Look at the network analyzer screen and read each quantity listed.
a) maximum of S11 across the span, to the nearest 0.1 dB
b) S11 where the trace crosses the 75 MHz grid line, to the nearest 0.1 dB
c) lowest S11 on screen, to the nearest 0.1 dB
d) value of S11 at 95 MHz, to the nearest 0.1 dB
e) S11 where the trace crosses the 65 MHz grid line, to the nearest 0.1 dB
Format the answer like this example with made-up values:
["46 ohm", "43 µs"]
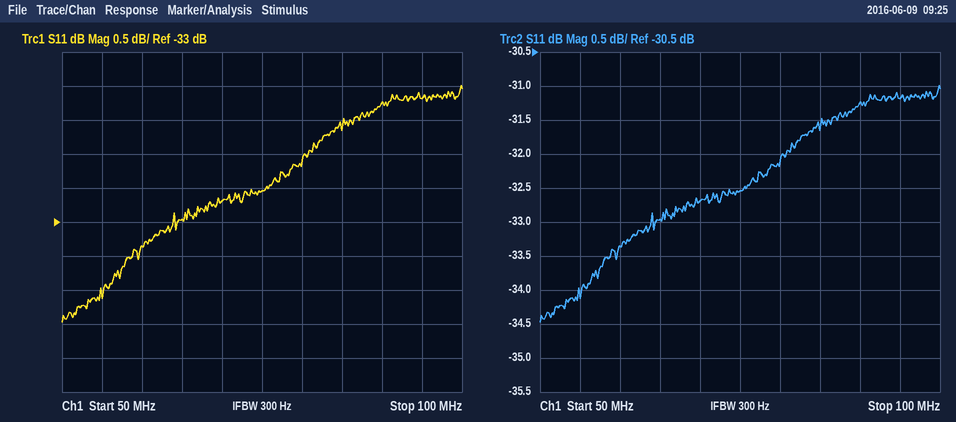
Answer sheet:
["-31.0 dB", "-32.5 dB", "-34.5 dB", "-31.2 dB", "-33.0 dB"]
